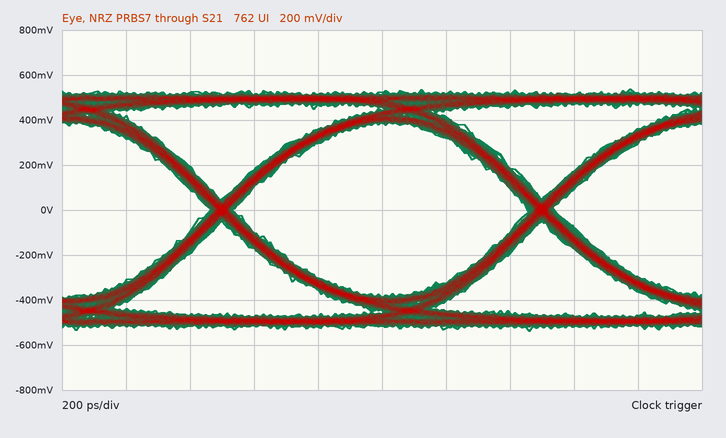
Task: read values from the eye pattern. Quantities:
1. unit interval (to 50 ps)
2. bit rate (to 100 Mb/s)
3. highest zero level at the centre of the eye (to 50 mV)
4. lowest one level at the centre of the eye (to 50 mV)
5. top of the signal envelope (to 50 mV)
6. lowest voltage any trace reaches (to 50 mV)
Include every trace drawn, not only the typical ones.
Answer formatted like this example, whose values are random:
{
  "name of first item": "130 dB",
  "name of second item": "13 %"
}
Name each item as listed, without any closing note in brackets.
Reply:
{
  "unit interval": "1.00 ns",
  "bit rate": "1.0 Gb/s",
  "highest zero level at the centre of the eye": "-400 mV",
  "lowest one level at the centre of the eye": "400 mV",
  "top of the signal envelope": "550 mV",
  "lowest voltage any trace reaches": "-550 mV"
}
